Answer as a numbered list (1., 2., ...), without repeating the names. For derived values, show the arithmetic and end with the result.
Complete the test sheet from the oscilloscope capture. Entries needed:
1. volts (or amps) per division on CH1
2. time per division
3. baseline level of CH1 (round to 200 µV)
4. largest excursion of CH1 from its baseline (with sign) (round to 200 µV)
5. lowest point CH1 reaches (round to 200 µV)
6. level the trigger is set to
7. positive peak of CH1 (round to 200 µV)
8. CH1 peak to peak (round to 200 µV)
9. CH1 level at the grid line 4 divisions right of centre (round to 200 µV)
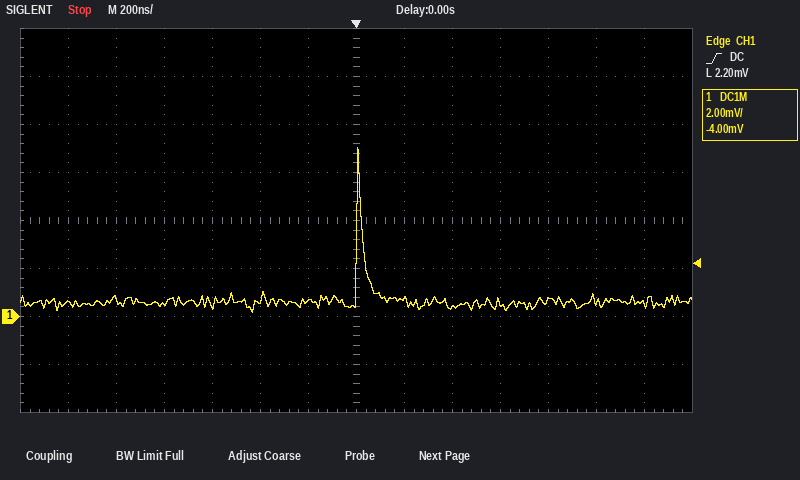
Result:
1. 2 mV
2. 200 ns
3. 600 µV
4. 7.0 mV − (600 µV) = +6.4 mV
5. 200 µV
6. 2.20 mV
7. 7.0 mV
8. 7.0 mV − (200 µV) = 6.8 mV
9. 600 µV
